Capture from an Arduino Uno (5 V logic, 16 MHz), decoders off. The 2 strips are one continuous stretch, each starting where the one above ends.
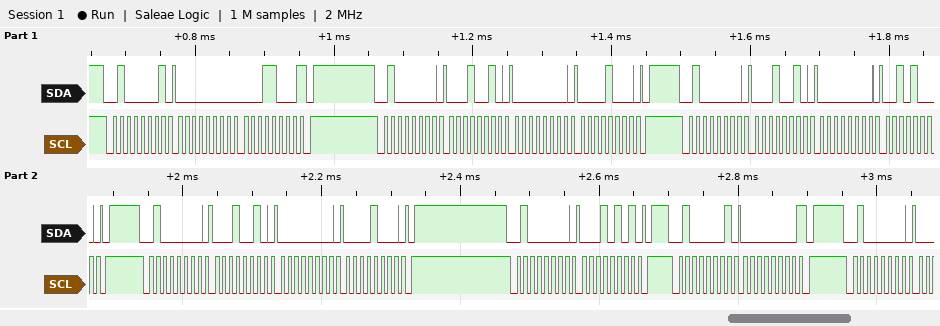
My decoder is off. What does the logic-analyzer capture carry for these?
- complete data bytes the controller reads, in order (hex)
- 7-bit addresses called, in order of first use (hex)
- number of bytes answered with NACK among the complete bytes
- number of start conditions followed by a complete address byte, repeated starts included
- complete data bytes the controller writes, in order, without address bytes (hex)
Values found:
00 18 00
0x20
2
7
12 00 08 12 00 28 12 00 08 15
